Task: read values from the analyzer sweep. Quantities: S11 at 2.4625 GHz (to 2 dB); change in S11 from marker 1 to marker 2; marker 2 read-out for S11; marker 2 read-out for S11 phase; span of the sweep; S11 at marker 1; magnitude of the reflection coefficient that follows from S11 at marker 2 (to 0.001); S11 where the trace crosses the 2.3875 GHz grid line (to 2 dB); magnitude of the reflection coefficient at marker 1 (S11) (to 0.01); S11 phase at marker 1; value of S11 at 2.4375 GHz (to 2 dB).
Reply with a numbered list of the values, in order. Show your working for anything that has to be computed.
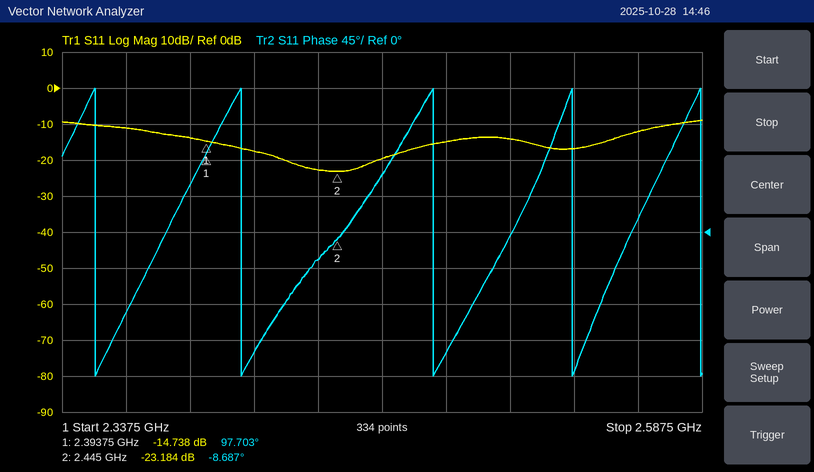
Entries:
1. -20 dB
2. -23.184 − (-14.738) = -8.446 dB
3. -23.184 dB
4. -8.687°
5. 250 MHz
6. -14.738 dB
7. 10^(-23.184/20) ≈ 0.069
8. -14 dB
9. 10^(-14.738/20) ≈ 0.18
10. 97.703°
11. -22 dB
